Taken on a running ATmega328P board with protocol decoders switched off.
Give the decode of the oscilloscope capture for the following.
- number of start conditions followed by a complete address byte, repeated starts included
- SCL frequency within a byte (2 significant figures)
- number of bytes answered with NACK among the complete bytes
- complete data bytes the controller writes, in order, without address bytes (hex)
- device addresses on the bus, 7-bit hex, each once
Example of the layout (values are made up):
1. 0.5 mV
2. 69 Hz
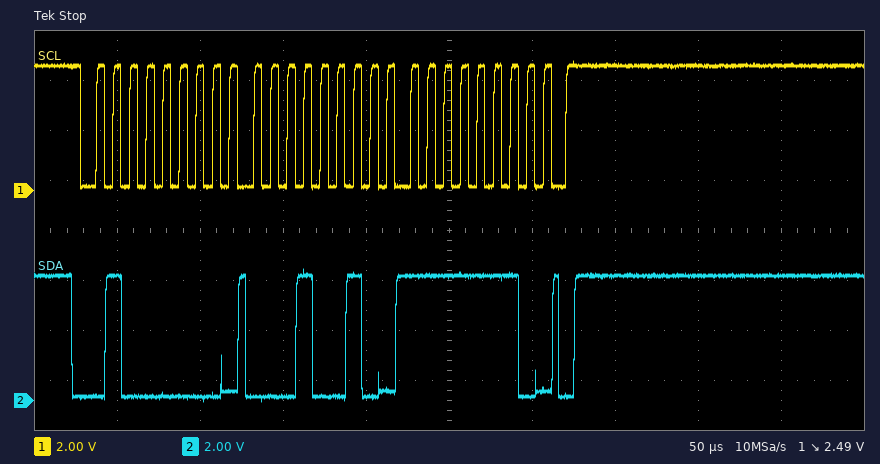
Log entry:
1. 1
2. 100 kHz
3. 0
4. 12 FE
5. 0x20
